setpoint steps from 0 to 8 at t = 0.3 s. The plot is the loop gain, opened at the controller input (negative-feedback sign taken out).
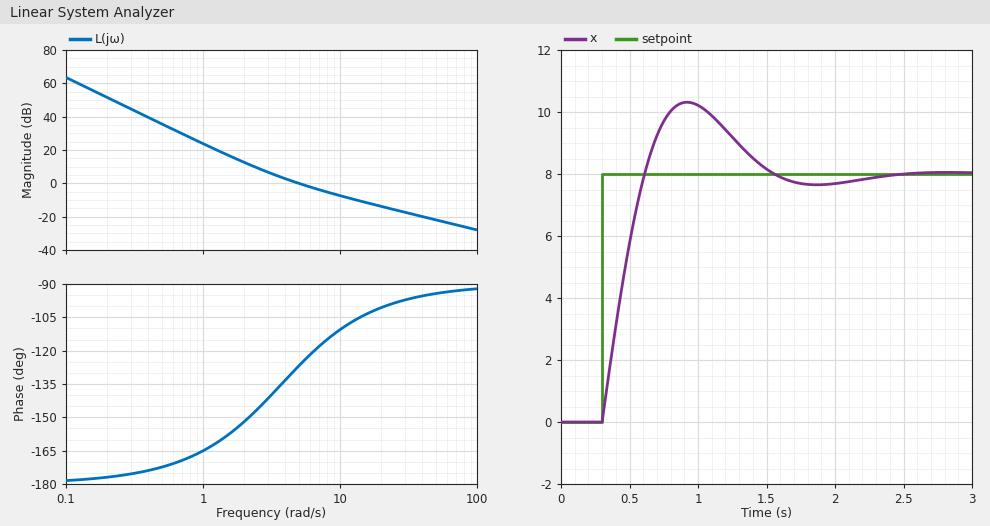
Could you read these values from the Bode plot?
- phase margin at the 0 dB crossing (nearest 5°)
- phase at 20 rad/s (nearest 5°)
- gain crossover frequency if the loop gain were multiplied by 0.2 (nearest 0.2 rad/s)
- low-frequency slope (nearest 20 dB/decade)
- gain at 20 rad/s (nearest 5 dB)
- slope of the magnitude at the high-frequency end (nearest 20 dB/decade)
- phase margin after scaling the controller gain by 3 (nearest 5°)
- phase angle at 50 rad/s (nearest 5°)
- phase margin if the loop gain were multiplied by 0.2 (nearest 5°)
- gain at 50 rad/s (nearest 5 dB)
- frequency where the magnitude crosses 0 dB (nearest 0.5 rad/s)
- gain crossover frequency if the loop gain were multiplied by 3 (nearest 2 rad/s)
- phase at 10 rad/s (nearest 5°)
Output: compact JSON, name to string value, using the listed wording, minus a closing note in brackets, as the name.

{"phase margin at the 0 dB crossing": "55°", "phase at 20 rad/s": "-100°", "gain crossover frequency if the loop gain were multiplied by 0.2": "1.8 rad/s", "low-frequency slope": "-40 dB/decade", "gain at 20 rad/s": "-15 dB", "slope of the magnitude at the high-frequency end": "-20 dB/decade", "phase margin after scaling the controller gain by 3": "75°", "phase angle at 50 rad/s": "-95°", "phase margin if the loop gain were multiplied by 0.2": "25°", "gain at 50 rad/s": "-20 dB", "frequency where the magnitude crosses 0 dB": "5.0 rad/s", "gain crossover frequency if the loop gain were multiplied by 3": "12 rad/s", "phase at 10 rad/s": "-110°"}
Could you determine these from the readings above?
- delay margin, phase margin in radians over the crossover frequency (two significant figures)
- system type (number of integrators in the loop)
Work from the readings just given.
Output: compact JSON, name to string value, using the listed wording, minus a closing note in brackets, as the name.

{"delay margin, phase margin in radians over the crossover frequency": "0.19 s", "system type": "2"}
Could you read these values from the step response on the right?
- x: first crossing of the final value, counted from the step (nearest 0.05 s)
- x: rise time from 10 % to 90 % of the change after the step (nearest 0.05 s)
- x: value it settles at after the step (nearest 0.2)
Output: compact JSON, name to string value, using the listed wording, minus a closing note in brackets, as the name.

{"x: first crossing of the final value, counted from the step": "0.30 s", "x: rise time from 10 % to 90 % of the change after the step": "0.25 s", "x: value it settles at after the step": "8.0"}
